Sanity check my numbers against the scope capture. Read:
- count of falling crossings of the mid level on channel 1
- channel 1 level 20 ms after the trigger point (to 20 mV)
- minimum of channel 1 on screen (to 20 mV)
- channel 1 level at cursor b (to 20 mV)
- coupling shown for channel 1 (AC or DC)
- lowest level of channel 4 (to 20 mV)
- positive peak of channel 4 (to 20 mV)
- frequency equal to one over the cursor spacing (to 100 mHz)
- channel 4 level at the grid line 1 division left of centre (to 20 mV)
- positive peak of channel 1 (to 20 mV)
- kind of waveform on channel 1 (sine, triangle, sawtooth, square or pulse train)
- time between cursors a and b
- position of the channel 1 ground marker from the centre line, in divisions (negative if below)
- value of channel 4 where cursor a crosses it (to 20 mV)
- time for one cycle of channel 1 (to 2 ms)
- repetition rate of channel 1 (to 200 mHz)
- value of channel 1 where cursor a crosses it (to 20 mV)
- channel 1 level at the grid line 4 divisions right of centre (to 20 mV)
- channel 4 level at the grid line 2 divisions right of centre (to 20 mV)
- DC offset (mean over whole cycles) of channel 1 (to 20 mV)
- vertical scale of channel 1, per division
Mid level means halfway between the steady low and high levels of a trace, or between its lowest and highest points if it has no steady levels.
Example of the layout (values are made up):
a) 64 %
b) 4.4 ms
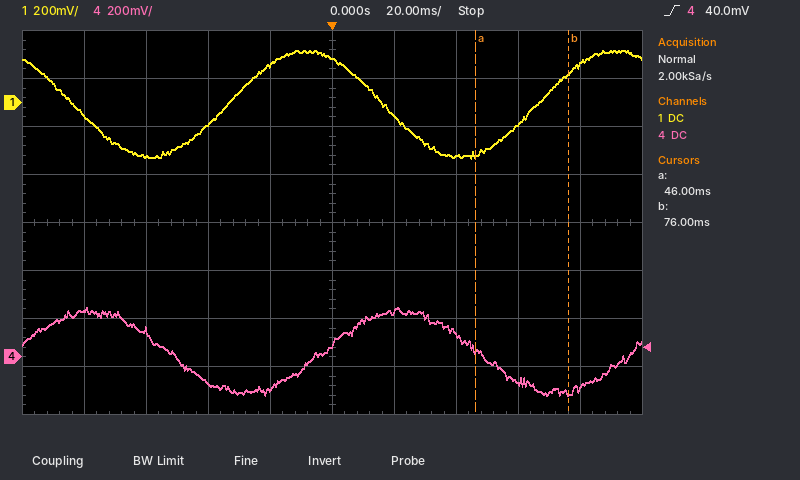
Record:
a) 2
b) -60 mV
c) -240 mV
d) 120 mV
e) DC
f) -160 mV
g) 200 mV
h) 33.3 Hz
i) -140 mV
j) 220 mV
k) sine
l) 30 ms
m) +2.5 div
n) 40 mV
o) 100 ms
p) 10.0 Hz
q) -220 mV
r) 160 mV
s) 100 mV
t) 0 mV
u) 200 mV
